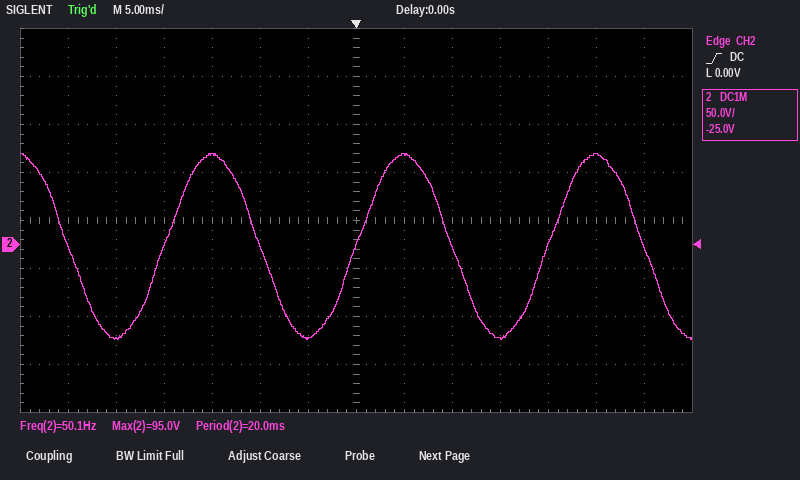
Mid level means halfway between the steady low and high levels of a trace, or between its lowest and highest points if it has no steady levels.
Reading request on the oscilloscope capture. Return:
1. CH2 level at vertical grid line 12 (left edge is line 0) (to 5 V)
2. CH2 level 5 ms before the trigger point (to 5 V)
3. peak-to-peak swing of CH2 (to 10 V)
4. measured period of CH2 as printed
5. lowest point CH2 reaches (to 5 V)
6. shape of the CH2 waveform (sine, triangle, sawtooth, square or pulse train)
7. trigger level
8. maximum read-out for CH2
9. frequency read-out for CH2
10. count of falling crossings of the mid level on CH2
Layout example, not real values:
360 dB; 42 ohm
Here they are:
95 V; -100 V; 190 V; 20.0 ms; -100 V; sine; 0.00 V; 95.0 V; 50.1 Hz; 4
